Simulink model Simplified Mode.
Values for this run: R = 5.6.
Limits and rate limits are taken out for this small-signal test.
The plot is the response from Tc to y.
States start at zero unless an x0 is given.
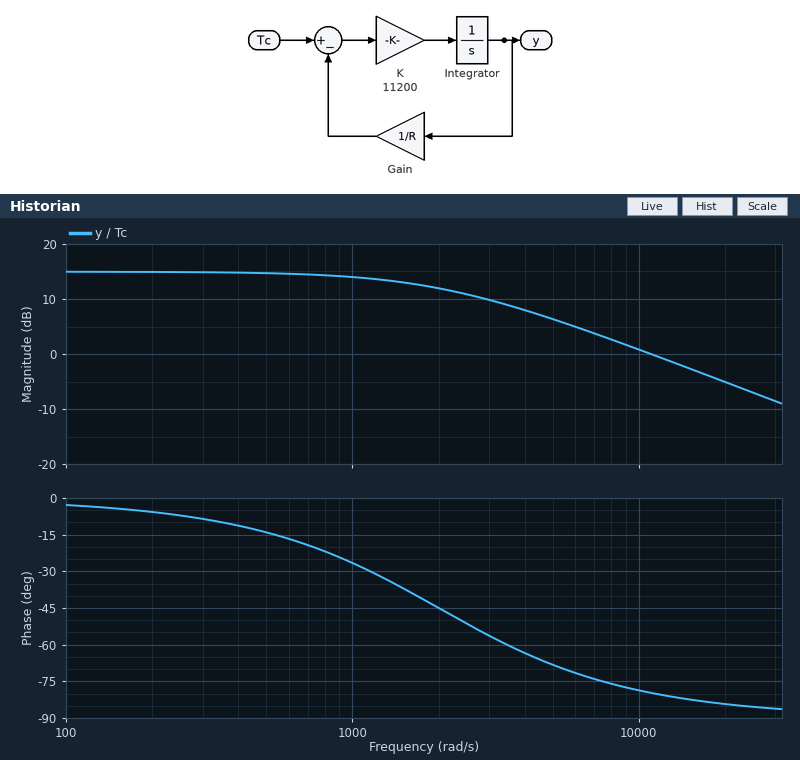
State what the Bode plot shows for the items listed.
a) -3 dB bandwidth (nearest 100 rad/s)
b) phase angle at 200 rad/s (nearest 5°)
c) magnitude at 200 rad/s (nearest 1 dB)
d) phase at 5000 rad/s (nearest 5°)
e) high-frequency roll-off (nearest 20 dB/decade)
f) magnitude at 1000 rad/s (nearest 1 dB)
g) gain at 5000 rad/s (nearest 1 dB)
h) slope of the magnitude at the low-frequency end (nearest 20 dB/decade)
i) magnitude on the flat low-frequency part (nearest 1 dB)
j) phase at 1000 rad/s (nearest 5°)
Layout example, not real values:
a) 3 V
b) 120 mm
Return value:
a) 2000 rad/s
b) -5°
c) 15 dB
d) -70°
e) -20 dB/decade
f) 14 dB
g) 6 dB
h) 0 dB/decade
i) 15 dB
j) -25°
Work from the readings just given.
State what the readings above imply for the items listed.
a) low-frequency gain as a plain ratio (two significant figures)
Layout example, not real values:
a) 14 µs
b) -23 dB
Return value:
a) 5.6
